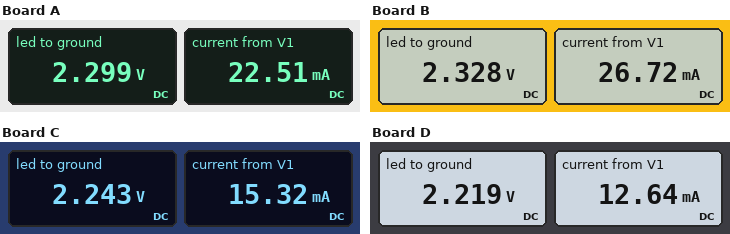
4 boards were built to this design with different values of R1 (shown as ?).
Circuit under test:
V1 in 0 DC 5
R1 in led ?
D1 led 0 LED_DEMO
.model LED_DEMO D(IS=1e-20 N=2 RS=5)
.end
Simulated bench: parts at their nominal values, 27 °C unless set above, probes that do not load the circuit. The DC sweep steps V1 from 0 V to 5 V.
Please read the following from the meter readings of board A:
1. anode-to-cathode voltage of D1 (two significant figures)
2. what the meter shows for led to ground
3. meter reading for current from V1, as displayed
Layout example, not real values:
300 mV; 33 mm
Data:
2.3 V; 2.299 V; 22.51 mA
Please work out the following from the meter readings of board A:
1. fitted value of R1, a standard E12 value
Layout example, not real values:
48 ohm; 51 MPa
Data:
120 Ω
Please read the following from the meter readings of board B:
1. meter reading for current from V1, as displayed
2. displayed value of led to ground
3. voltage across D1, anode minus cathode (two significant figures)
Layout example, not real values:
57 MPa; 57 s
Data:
26.72 mA; 2.328 V; 2.3 V
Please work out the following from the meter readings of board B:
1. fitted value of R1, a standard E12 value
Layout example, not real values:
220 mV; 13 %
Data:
100 Ω
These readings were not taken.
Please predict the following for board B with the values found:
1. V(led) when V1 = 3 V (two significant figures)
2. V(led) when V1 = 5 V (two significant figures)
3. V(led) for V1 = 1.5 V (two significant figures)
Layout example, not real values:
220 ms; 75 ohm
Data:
2.2 V; 2.3 V; 1.5 V
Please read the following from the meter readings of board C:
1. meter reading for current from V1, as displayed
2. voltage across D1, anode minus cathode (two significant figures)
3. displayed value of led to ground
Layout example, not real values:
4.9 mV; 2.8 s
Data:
15.32 mA; 2.2 V; 2.243 V
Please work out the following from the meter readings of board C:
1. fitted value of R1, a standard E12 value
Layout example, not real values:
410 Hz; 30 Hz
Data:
180 Ω
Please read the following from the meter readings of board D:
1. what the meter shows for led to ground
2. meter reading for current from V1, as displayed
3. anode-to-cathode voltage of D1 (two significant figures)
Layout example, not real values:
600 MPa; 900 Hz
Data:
2.219 V; 12.64 mA; 2.2 V
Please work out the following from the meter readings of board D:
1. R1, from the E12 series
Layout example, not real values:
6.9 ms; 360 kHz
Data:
220 Ω
